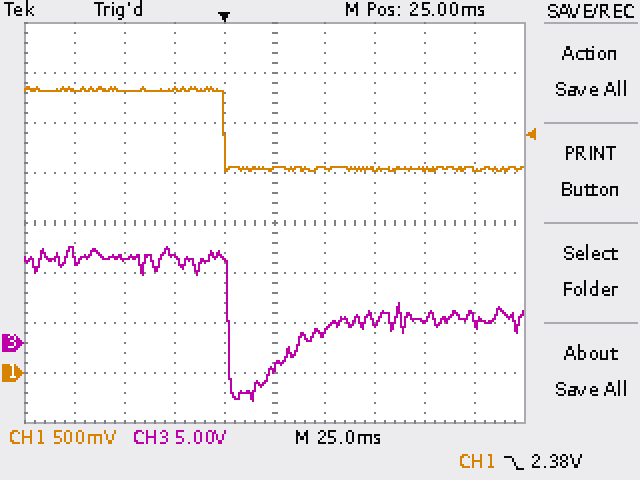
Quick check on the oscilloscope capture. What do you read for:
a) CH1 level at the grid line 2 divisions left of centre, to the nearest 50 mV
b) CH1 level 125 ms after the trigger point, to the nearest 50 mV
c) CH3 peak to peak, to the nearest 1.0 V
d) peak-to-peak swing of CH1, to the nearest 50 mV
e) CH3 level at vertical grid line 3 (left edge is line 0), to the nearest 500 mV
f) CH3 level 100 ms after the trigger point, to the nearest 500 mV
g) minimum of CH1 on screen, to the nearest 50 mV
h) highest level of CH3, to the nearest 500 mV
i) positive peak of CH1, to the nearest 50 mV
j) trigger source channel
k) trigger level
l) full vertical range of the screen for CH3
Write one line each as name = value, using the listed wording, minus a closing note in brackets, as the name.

CH1 level at the grid line 2 divisions left of centre, to the nearest 50 mV = 2.85 V
CH1 level 125 ms after the trigger point, to the nearest 50 mV = 2.05 V
CH3 peak to peak, to the nearest 1.0 V = 15.0 V
peak-to-peak swing of CH1, to the nearest 50 mV = 850 mV
CH3 level at vertical grid line 3 (left edge is line 0), to the nearest 500 mV = 8.5 V
CH3 level 100 ms after the trigger point, to the nearest 500 mV = 2.5 V
minimum of CH1 on screen, to the nearest 50 mV = 2.00 V
highest level of CH3, to the nearest 500 mV = 9.5 V
positive peak of CH1, to the nearest 50 mV = 2.85 V
trigger source channel = CH1
trigger level = 2.38 V
full vertical range of the screen for CH3 = 40 V
